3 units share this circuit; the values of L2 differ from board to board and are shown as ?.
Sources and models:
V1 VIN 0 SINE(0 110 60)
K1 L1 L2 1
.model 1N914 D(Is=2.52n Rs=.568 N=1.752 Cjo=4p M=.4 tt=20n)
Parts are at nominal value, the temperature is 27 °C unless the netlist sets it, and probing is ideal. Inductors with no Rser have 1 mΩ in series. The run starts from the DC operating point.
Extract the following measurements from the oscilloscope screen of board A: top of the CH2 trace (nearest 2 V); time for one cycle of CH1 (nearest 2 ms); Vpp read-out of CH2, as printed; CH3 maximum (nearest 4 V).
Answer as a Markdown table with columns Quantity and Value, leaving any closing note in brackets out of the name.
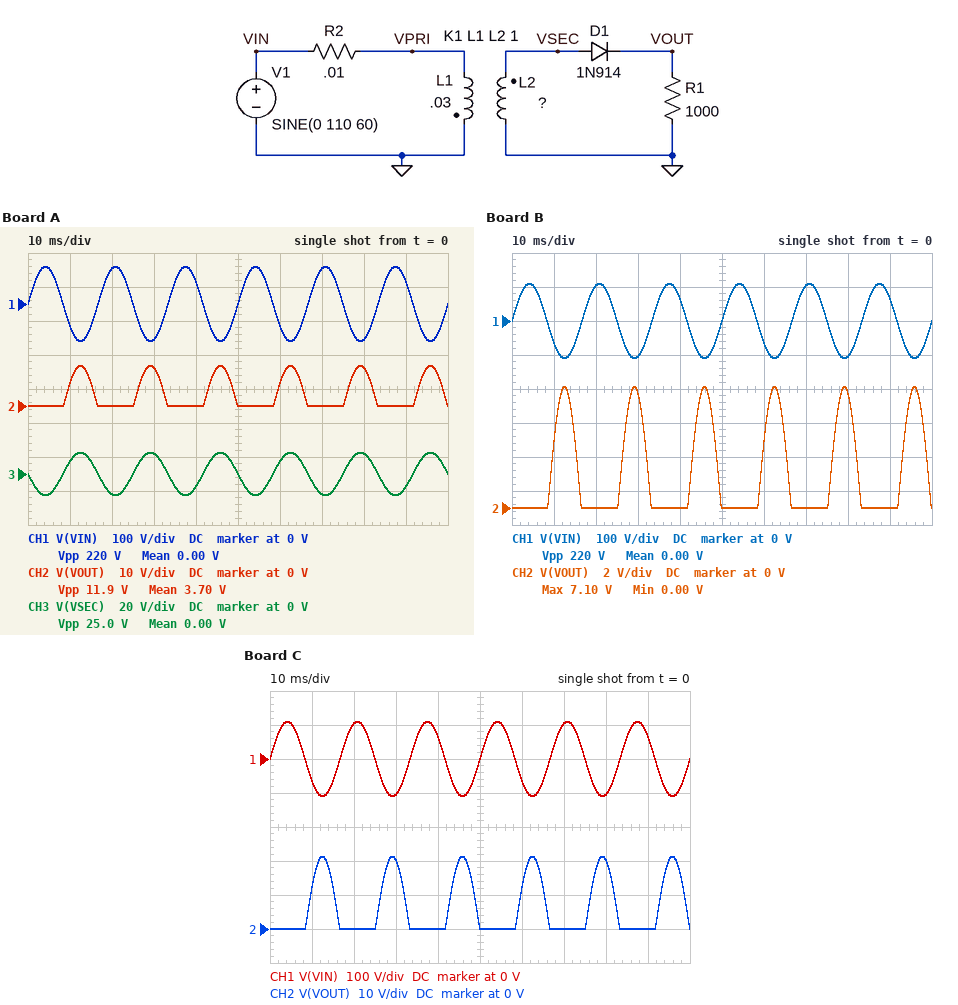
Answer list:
| Quantity | Value |
|---|---|
| top of the CH2 trace | 12 V |
| time for one cycle of CH1 | 16 ms |
| Vpp read-out of CH2, as printed | 11.9 V |
| CH3 maximum | 12 V |
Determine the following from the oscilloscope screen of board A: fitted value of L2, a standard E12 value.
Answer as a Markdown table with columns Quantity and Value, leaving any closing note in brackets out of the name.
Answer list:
| Quantity | Value |
|---|---|
| fitted value of L2, a standard E12 value | 390 µH |
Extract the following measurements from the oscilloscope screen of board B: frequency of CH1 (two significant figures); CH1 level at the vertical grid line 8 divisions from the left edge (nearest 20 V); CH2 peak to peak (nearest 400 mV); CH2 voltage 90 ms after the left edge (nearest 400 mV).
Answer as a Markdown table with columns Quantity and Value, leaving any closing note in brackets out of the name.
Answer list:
| Quantity | Value |
|---|---|
| frequency of CH1 | 60 Hz |
| CH1 level at the vertical grid line 8 divisions from the left edge | -100 V |
| CH2 peak to peak | 7.2 V |
| CH2 voltage 90 ms after the left edge | 0 V |
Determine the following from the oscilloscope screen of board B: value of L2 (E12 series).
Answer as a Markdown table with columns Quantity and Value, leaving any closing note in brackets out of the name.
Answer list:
| Quantity | Value |
|---|---|
| value of L2 | 150 µH |
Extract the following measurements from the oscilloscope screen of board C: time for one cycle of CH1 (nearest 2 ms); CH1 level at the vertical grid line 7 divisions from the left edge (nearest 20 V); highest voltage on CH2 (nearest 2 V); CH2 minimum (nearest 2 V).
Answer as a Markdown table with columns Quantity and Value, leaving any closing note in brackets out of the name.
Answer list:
| Quantity | Value |
|---|---|
| time for one cycle of CH1 | 16 ms |
| CH1 level at the vertical grid line 7 divisions from the left edge | 100 V |
| highest voltage on CH2 | 22 V |
| CH2 minimum | 0 V |
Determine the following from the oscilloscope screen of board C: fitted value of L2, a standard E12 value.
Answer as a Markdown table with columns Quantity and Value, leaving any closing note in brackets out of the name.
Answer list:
| Quantity | Value |
|---|---|
| fitted value of L2, a standard E12 value | 1.2 mH |
